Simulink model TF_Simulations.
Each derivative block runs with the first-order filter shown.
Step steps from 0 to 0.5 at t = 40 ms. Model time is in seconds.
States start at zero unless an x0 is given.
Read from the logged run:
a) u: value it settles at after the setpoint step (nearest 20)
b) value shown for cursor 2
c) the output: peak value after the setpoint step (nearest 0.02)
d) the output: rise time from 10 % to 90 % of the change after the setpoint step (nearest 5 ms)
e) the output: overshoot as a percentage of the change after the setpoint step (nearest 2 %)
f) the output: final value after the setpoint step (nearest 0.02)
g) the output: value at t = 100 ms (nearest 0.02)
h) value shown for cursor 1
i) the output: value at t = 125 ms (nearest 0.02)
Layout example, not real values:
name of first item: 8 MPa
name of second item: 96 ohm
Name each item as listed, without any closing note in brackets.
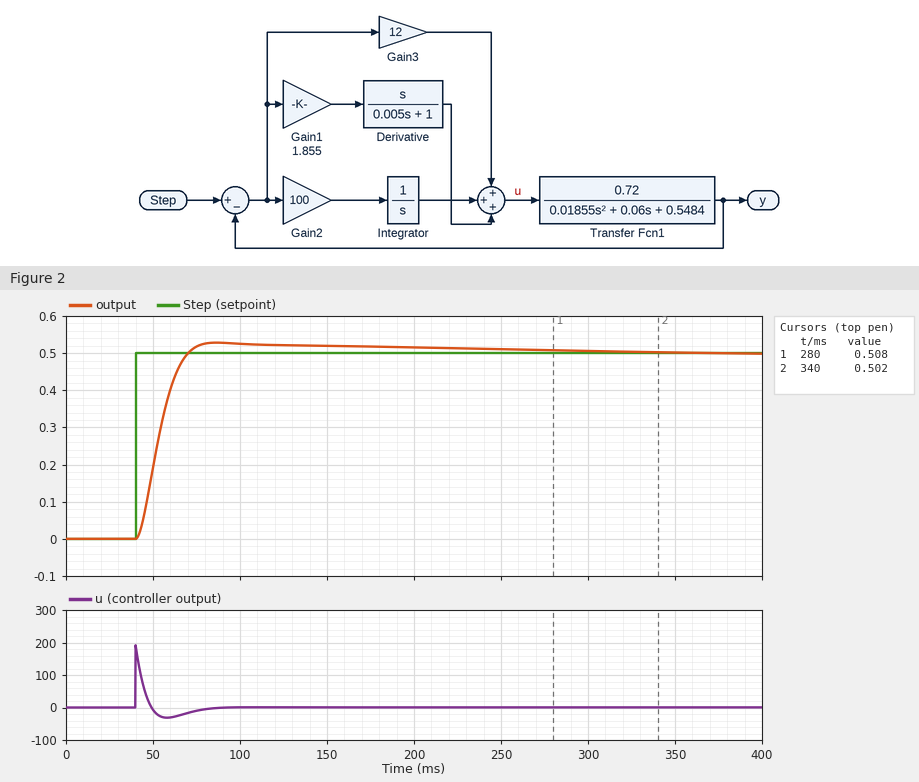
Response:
u: value it settles at after the setpoint step: 0
value shown for cursor 2: 0.502
the output: peak value after the setpoint step: 0.52
the output: rise time from 10 % to 90 % of the change after the setpoint step: 20 ms
the output: overshoot as a percentage of the change after the setpoint step: 6 %
the output: final value after the setpoint step: 0.50
the output: value at t = 100 ms: 0.52
value shown for cursor 1: 0.508
the output: value at t = 125 ms: 0.52
